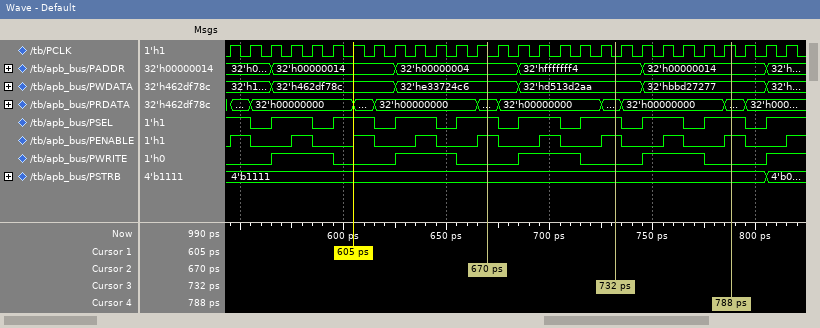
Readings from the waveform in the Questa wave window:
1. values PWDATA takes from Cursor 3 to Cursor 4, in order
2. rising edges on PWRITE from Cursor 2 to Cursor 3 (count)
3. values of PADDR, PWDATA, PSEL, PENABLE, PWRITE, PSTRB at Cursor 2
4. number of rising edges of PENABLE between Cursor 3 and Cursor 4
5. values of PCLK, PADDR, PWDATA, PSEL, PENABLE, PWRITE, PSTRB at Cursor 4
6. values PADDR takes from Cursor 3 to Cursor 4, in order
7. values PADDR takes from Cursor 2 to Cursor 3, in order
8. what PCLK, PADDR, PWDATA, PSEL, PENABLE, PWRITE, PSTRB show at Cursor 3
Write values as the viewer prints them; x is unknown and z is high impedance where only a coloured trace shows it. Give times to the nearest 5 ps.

32'hd513d2aa, 32'hbbd27277
1
PADDR=32'h00000004, PWDATA=32'he33724c6, PSEL=1, PENABLE=1, PWRITE=0, PSTRB=4'b1111
2
PCLK=1, PADDR=32'h00000014, PWDATA=32'hbbd27277, PSEL=1, PENABLE=1, PWRITE=0, PSTRB=4'b1111
32'hfffffff4, 32'h00000014
32'h00000004, 32'hfffffff4
PCLK=0, PADDR=32'hfffffff4, PWDATA=32'hd513d2aa, PSEL=1, PENABLE=1, PWRITE=0, PSTRB=4'b1111
